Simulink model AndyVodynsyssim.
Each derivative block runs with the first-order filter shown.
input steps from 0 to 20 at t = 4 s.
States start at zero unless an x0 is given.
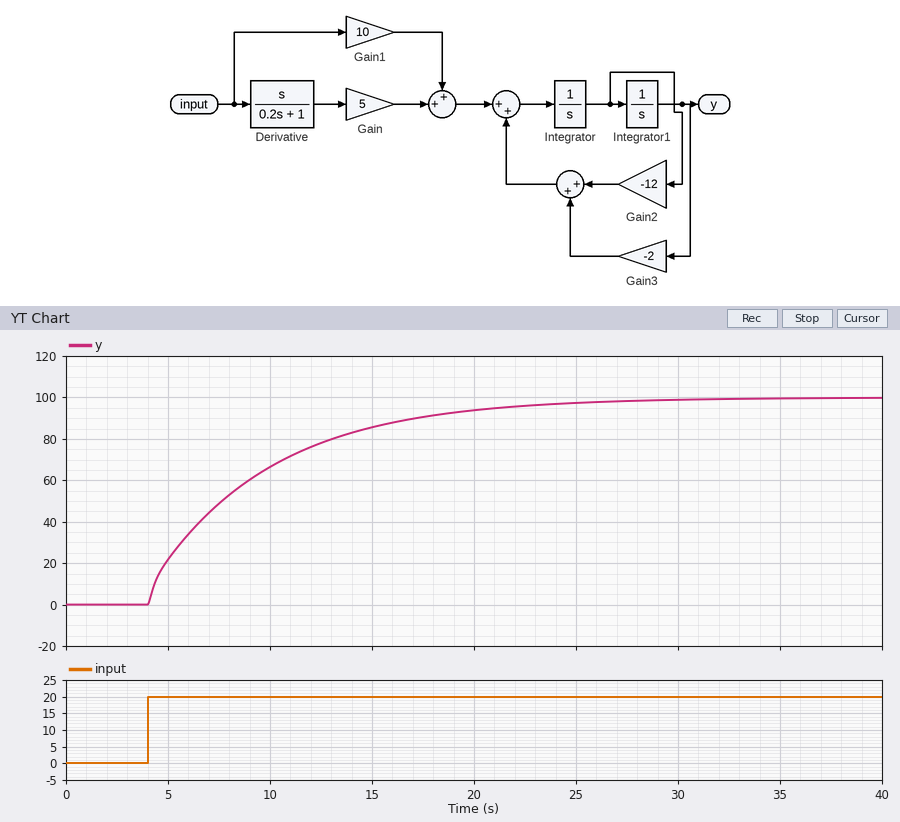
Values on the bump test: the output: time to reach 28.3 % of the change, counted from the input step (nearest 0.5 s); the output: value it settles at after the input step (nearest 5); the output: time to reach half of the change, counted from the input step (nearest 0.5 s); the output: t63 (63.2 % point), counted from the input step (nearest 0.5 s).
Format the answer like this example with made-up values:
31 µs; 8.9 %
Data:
1.5 s; 100; 3.5 s; 5.5 s
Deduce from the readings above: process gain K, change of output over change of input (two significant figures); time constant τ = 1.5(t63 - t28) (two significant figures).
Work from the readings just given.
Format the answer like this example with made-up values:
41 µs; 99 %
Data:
5.0; 6.0 s
